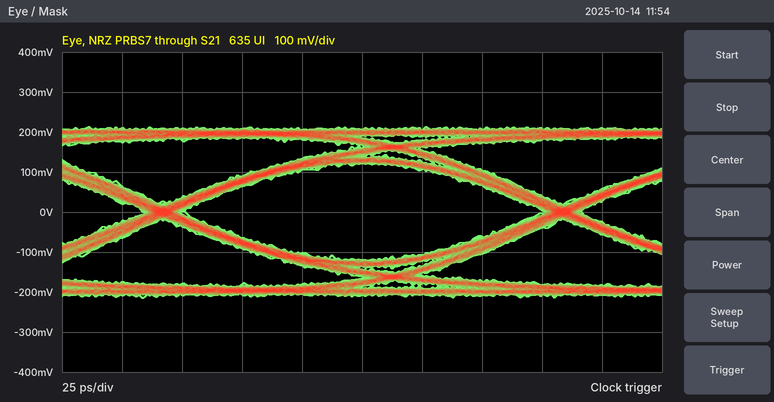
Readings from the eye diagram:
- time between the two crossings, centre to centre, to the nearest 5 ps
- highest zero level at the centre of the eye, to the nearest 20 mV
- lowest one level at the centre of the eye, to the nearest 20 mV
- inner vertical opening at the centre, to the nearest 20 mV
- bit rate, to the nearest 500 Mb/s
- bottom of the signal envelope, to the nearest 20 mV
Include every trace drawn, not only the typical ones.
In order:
165 ps
-120 mV
120 mV
240 mV
6.0 Gb/s
-220 mV
